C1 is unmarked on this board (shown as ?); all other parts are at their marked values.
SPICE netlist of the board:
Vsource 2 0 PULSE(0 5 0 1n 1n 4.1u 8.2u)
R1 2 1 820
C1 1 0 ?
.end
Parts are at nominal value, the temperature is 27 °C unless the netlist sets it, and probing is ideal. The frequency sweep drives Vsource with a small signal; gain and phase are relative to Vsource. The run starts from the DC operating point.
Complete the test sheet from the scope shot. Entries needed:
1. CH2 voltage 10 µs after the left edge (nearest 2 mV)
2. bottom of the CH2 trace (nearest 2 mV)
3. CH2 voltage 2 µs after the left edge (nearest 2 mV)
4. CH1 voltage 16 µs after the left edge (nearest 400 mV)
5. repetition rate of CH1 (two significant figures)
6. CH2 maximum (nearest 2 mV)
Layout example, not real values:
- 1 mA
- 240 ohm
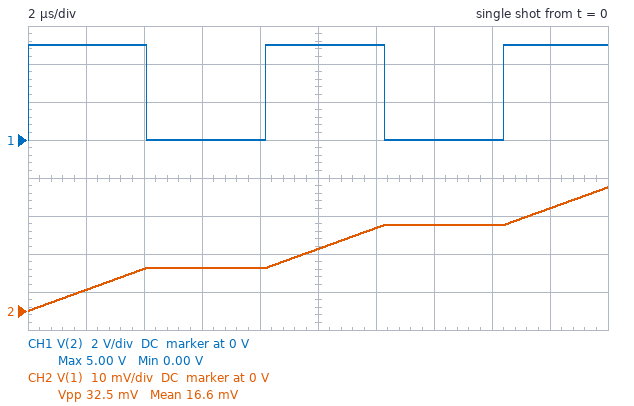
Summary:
- 16 mV
- 0 V
- 6 mV
- 0 V
- 120 kHz
- 32 mV
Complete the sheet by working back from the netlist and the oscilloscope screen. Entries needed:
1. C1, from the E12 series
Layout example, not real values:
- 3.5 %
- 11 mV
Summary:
- 2.2 µF
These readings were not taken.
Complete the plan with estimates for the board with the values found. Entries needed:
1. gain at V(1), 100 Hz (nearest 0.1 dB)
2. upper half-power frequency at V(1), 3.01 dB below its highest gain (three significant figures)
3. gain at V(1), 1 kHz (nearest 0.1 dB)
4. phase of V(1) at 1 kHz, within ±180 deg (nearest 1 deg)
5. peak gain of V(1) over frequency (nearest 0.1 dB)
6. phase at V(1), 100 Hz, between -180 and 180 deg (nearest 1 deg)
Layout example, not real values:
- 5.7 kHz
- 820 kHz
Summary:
- -3.6 dB
- 88.2 Hz
- -21.1 dB
- -85 deg
- 0 dB
- -49 deg
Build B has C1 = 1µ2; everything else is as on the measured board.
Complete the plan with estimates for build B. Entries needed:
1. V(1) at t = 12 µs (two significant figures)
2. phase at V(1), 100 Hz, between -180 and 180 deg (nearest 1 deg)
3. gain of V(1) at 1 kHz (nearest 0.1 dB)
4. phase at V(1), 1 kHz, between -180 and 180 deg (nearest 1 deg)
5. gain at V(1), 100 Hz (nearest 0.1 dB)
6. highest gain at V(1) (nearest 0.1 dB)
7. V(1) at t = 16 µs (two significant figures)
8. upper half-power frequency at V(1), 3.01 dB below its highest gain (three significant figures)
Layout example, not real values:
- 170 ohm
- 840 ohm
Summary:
- 40 mV
- -32 deg
- -15.9 dB
- -81 deg
- -1.4 dB
- 0 dB
- 41 mV
- 162 Hz
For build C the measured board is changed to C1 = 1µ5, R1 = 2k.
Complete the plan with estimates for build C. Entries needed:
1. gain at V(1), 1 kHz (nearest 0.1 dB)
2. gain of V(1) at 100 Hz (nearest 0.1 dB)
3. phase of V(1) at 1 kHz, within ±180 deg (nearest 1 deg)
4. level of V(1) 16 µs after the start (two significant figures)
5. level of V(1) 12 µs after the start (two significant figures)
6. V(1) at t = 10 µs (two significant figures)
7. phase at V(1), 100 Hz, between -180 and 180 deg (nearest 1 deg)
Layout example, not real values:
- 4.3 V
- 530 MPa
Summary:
- -25.5 dB
- -6.6 dB
- -87 deg
- 14 mV
- 13 mV
- 9.8 mV
- -62 deg
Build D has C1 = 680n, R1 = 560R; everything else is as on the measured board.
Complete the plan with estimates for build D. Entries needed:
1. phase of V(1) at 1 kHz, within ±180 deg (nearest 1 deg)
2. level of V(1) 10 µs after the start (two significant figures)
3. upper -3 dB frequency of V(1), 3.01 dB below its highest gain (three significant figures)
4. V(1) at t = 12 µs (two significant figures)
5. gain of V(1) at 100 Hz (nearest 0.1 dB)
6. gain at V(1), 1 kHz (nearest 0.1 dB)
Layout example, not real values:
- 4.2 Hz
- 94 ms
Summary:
- -67 deg
- 76 mV
- 418 Hz
- 100 mV
- -0.2 dB
- -8.3 dB
